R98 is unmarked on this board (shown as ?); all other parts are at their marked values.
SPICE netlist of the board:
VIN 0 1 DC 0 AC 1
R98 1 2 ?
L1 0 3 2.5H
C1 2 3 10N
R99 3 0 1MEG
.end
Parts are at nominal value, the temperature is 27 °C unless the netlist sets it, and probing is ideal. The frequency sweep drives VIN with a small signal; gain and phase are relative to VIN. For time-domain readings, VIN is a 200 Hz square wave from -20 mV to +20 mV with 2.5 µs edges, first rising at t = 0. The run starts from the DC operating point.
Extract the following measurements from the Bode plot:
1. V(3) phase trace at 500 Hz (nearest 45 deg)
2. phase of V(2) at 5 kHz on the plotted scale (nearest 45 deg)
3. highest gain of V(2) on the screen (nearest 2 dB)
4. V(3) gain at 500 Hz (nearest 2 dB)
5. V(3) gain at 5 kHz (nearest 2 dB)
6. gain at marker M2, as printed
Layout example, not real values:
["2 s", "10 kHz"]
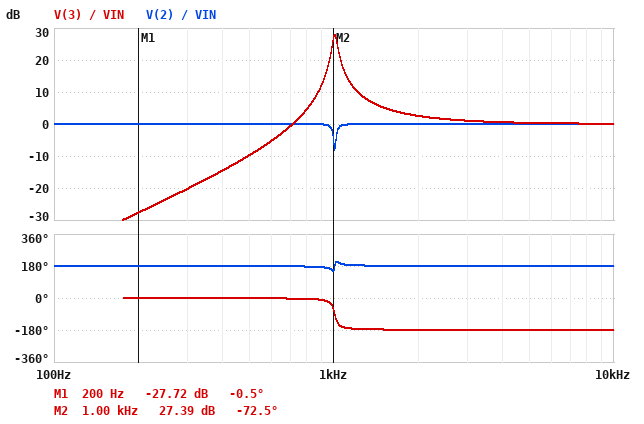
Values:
["0 deg", "180 deg", "0 dB", "-10 dB", "0 dB", "27.39 dB"]
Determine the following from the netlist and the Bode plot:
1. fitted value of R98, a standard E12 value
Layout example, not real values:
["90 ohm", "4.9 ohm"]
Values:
["390 Ω"]
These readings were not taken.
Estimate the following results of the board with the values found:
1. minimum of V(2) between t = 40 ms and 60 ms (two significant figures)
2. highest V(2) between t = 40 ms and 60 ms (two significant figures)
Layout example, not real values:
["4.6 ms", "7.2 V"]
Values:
["-23 mV", "23 mV"]
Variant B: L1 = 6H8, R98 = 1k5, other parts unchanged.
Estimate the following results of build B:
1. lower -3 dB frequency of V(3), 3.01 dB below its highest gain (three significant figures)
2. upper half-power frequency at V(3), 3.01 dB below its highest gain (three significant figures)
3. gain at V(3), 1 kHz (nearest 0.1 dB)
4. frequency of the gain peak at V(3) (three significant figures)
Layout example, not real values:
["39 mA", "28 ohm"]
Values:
["587 Hz", "638 Hz", "4.0 dB", "611 Hz"]
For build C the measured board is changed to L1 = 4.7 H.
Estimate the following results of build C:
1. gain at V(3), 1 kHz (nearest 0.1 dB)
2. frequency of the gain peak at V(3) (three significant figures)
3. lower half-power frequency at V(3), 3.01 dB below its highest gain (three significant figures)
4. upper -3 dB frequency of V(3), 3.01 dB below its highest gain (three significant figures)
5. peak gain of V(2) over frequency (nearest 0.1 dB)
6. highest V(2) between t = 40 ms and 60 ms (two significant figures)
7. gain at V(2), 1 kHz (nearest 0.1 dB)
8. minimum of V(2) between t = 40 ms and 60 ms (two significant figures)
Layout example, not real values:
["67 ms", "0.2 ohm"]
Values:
["6.7 dB", "734 Hz", "720 Hz", "749 Hz", "0 dB", "20 mV", "0 dB", "-20 mV"]
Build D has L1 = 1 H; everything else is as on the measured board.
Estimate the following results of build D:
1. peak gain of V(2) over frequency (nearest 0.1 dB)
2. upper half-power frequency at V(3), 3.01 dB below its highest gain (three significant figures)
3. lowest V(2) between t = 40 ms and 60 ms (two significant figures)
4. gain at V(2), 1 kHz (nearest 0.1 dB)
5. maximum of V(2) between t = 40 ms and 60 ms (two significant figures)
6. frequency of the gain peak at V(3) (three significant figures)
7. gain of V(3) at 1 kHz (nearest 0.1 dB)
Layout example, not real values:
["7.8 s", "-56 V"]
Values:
["0 dB", "1.63 kHz", "-21 mV", "0 dB", "21 mV", "1.59 kHz", "-3.7 dB"]
